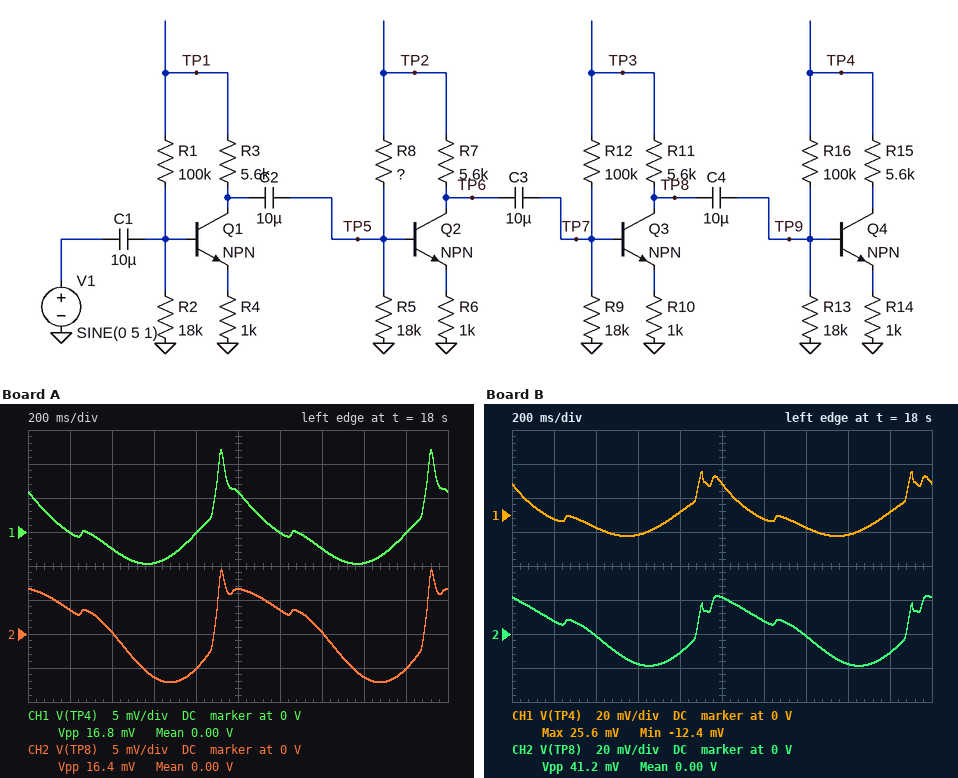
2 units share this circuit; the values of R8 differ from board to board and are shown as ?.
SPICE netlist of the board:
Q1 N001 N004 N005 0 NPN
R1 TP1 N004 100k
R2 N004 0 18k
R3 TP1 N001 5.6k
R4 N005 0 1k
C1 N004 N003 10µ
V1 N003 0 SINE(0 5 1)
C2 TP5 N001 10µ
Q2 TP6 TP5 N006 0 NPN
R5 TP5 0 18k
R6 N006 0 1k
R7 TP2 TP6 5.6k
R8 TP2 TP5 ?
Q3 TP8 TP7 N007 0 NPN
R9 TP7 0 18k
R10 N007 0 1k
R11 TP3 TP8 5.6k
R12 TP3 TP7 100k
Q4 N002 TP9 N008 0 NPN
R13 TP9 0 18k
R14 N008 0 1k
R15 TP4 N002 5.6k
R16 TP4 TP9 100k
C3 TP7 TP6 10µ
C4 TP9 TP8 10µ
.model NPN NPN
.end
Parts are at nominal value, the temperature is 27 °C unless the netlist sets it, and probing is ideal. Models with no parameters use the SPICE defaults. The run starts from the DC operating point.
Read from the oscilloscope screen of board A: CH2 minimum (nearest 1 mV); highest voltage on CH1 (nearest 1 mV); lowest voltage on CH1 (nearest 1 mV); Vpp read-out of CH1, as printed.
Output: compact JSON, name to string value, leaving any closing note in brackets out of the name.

{"CH2 minimum": "-7 mV", "highest voltage on CH1": "12 mV", "lowest voltage on CH1": "-5 mV", "Vpp read-out of CH1, as printed": "16.8 mV"}
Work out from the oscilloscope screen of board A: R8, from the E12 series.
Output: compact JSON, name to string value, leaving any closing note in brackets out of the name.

{"R8, from the E12 series": "180 kΩ"}
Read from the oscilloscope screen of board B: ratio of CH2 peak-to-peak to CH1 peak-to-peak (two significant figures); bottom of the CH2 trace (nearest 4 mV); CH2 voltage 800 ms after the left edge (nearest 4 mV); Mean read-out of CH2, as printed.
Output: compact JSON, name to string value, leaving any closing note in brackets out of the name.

{"ratio of CH2 peak-to-peak to CH1 peak-to-peak": "1.1", "bottom of the CH2 trace": "-20 mV", "CH2 voltage 800 ms after the left edge": "-12 mV", "Mean read-out of CH2, as printed": "0.00 V"}
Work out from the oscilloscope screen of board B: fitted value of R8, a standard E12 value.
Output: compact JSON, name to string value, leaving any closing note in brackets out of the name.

{"fitted value of R8, a standard E12 value": "39 kΩ"}
